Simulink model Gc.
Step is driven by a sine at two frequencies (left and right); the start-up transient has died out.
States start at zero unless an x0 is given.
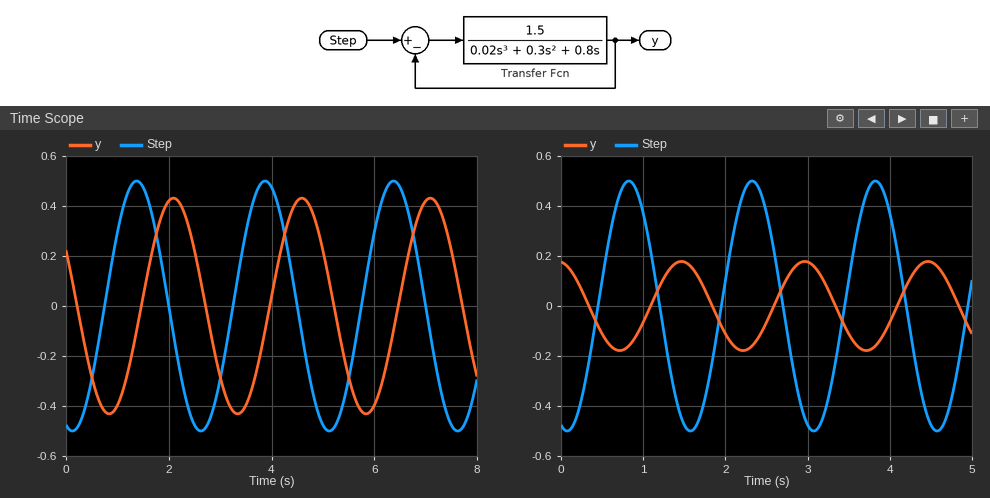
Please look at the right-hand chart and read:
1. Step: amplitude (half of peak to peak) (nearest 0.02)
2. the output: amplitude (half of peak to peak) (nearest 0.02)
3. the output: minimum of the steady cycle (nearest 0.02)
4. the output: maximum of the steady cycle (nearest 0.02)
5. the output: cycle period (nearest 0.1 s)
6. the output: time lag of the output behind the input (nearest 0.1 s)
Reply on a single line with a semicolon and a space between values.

0.50; 0.18; -0.18; 0.18; 1.5 s; 0.6 s
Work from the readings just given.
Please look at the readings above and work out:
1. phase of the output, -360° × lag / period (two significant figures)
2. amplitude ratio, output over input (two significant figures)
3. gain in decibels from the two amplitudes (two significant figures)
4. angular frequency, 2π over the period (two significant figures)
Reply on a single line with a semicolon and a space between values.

-140°; 0.36; -8.9 dB; 4.2 rad/s
